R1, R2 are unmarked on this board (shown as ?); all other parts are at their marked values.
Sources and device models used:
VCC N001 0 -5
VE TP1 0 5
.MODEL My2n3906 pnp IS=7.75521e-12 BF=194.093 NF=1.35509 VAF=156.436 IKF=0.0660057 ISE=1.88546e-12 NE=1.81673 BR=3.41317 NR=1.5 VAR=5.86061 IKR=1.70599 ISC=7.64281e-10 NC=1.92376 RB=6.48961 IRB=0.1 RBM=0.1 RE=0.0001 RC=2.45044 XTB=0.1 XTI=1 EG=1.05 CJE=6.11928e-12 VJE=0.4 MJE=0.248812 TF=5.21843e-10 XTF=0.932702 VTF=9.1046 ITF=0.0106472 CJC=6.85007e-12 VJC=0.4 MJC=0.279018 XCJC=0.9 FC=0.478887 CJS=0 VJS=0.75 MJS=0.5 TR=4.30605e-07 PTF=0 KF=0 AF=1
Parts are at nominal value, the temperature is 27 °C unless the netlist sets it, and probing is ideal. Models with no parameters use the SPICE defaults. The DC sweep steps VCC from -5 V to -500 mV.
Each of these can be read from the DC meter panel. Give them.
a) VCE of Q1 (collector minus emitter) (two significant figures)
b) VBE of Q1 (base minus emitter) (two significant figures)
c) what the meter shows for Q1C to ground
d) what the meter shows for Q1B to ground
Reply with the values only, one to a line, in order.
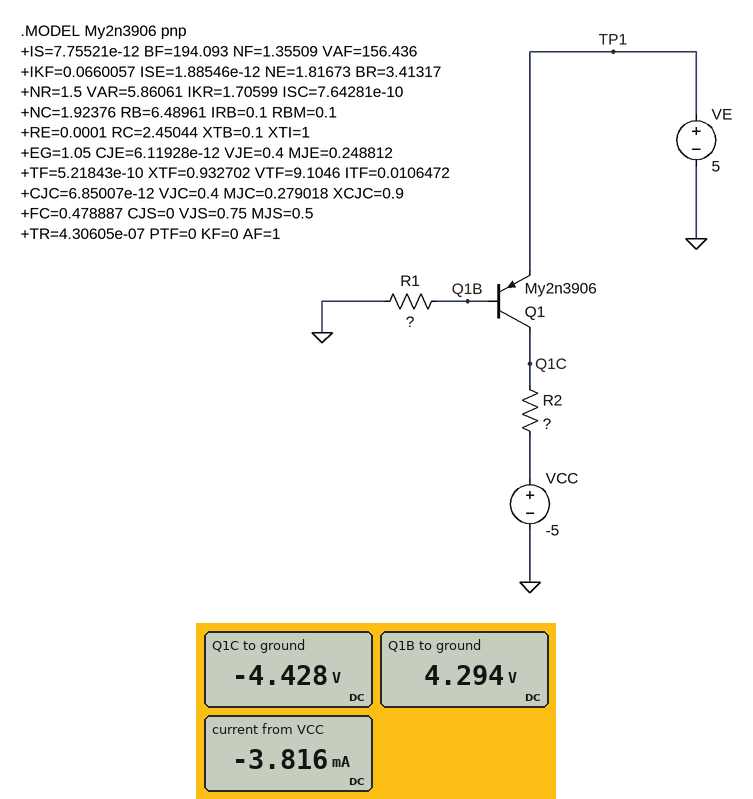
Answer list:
-9.4 V
-710 mV
-4.428 V
4.294 V
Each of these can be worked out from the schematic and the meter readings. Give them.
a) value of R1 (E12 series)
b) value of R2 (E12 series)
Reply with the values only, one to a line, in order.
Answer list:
150 kΩ
150 Ω
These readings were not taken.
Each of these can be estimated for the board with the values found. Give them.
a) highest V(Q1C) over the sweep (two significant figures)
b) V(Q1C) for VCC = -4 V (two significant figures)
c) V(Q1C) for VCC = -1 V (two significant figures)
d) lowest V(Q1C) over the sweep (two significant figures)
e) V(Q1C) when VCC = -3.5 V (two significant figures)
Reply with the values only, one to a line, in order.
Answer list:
55 mV
-3.4 V
-440 mV
-4.4 V
-2.9 V
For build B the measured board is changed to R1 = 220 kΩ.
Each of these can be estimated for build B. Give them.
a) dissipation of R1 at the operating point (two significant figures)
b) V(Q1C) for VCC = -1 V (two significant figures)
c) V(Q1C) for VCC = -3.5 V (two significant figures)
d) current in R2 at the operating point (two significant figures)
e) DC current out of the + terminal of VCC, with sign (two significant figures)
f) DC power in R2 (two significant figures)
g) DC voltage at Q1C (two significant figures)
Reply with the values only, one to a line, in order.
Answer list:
84 µW
-620 mV
-3.1 V
2.6 mA
-2.6 mA
1.0 mW
-4.6 V
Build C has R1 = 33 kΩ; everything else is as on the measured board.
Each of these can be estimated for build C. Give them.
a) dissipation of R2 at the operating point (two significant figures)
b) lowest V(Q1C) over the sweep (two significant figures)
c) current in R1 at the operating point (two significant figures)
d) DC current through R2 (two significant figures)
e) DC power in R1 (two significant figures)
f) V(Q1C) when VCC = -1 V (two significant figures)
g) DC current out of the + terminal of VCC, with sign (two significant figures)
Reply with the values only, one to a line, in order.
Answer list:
35 mW
-2.7 V
130 µA
15 mA
540 µW
1.2 V
-15 mA
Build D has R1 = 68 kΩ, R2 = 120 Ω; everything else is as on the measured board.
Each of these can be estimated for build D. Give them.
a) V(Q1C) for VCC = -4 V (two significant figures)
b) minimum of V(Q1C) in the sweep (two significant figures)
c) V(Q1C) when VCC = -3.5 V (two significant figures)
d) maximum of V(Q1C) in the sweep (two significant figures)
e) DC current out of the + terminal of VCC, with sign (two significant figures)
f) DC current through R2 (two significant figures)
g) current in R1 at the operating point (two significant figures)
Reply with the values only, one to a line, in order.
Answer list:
-3.0 V
-4.0 V
-2.5 V
440 mV
-8.1 mA
8.1 mA
63 µA
